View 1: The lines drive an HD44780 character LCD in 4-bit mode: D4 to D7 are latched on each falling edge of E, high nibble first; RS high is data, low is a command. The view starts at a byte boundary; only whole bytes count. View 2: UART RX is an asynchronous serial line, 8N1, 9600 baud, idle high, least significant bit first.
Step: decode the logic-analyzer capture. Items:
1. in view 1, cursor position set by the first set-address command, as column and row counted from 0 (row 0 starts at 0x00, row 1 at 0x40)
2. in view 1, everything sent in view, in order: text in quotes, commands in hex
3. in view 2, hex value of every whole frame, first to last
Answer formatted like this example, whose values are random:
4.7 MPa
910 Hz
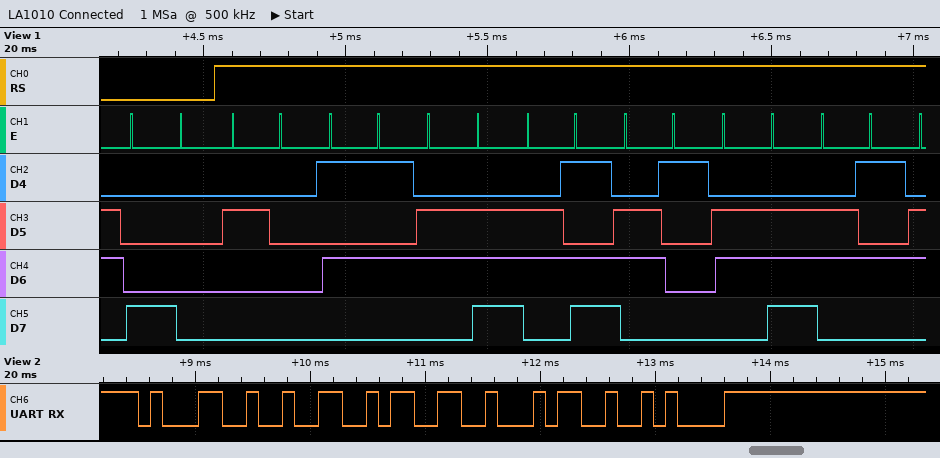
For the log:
column 0, row 0
0x80 " Unmane"
0x31 0x32 0x33 0x34 0x0A
